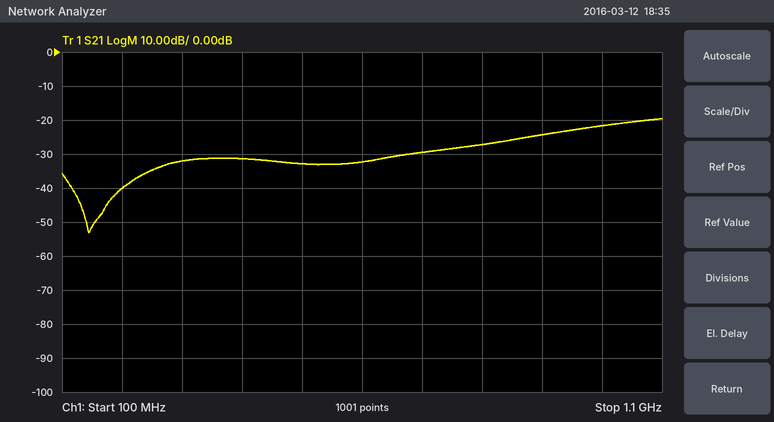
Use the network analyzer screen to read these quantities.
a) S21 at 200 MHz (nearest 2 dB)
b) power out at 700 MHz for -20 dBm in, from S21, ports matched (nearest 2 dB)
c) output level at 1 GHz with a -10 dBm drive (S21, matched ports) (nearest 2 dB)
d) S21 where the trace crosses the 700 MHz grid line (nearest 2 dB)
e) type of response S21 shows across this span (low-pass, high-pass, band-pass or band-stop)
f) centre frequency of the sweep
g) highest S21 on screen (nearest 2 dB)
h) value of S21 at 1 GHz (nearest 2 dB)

-40 dB
-50 dBm
-32 dBm
-30 dB
high-pass
600 MHz
-20 dB
-22 dB
